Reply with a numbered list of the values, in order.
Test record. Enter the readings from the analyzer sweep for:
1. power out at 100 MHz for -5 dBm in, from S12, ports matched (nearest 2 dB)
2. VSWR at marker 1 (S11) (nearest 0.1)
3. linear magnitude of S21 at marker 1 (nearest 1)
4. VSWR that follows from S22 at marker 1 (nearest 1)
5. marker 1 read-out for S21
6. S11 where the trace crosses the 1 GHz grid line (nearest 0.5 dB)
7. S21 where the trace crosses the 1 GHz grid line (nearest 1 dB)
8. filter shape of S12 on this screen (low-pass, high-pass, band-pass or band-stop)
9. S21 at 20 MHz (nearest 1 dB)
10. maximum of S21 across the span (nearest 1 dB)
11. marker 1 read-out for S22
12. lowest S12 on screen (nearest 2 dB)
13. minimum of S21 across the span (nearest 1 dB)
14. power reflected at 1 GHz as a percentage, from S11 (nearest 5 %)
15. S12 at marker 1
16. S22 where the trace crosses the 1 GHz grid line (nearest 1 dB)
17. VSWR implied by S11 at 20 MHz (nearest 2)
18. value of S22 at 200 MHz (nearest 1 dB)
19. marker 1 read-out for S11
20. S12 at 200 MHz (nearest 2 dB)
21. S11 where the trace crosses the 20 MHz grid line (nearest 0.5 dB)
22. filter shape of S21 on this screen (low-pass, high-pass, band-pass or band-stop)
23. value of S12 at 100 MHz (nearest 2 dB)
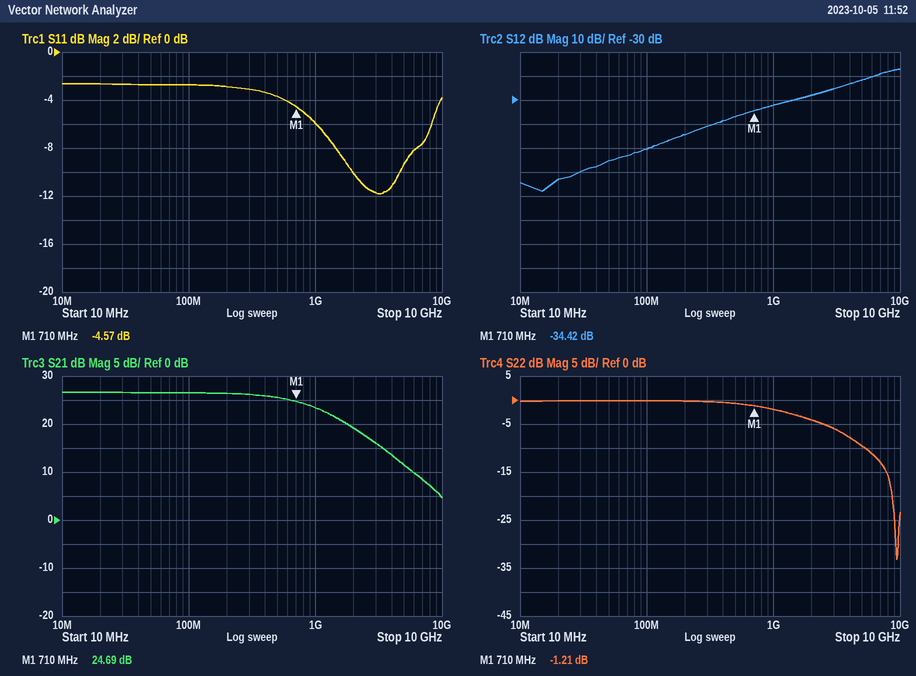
1. -56 dBm
2. 3.9
3. 17
4. 14
5. 24.69 dB
6. -6.0 dB
7. 23 dB
8. high-pass
9. 27 dB
10. 27 dB
11. -1.21 dB
12. -68 dB
13. 5 dB
14. 25 %
15. -34.42 dB
16. -2 dB
17. 6
18. 0 dB
19. -4.57 dB
20. -44 dB
21. -2.5 dB
22. low-pass
23. -50 dB
